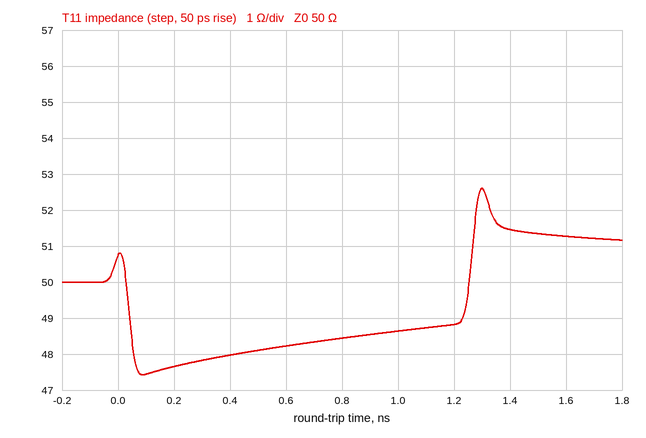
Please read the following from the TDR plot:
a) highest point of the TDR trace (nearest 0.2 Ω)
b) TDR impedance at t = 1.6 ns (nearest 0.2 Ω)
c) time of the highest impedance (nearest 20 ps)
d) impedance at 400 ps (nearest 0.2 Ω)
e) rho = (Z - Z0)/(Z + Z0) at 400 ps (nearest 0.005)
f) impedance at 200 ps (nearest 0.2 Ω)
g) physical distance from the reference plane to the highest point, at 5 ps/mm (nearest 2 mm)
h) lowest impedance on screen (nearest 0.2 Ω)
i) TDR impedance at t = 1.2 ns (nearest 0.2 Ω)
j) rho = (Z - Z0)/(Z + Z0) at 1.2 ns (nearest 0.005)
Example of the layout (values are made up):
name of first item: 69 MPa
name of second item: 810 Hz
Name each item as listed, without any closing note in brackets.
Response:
highest point of the TDR trace: 52.6 Ω
TDR impedance at t = 1.6 ns: 51.2 Ω
time of the highest impedance: 1.30 ns
impedance at 400 ps: 48.0 Ω
rho = (Z - Z0)/(Z + Z0) at 400 ps: -0.020
impedance at 200 ps: 47.6 Ω
physical distance from the reference plane to the highest point, at 5 ps/mm: 130 mm
lowest impedance on screen: 47.4 Ω
TDR impedance at t = 1.2 ns: 48.8 Ω
rho = (Z - Z0)/(Z + Z0) at 1.2 ns: -0.010
